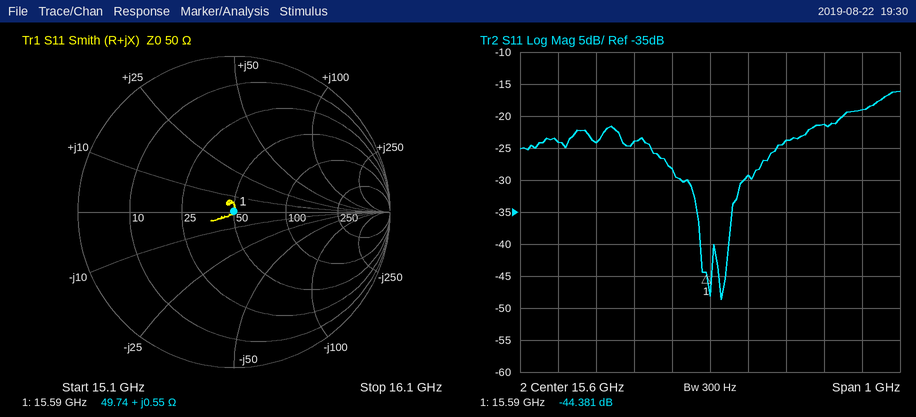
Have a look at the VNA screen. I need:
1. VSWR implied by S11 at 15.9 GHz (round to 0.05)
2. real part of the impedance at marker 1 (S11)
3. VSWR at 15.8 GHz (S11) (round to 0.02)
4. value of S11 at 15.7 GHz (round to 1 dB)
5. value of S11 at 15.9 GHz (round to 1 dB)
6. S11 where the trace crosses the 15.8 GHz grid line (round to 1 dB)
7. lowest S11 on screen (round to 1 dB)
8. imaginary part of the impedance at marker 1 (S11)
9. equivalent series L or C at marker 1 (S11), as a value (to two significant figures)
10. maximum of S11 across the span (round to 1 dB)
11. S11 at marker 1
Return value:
1.20
49.74 Ω
1.14
-29 dB
-21 dB
-24 dB
-49 dB
+0.55 Ω
5.6 pH
-16 dB
-44.381 dB
